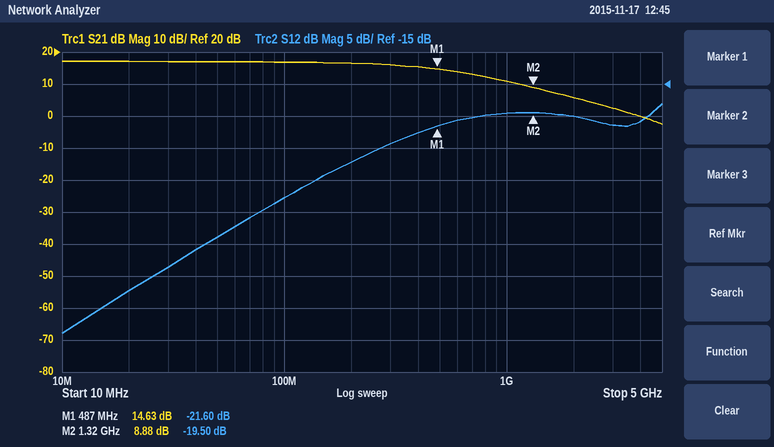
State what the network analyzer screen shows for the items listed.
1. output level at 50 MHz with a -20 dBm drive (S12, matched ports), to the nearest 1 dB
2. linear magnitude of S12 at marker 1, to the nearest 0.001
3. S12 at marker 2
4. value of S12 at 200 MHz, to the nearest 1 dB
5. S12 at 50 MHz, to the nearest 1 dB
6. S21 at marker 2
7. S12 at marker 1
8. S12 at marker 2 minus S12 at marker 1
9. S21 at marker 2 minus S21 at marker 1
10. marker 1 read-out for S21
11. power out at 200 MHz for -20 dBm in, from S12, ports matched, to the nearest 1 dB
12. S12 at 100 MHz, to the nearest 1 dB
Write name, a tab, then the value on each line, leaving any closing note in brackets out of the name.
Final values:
output level at 50 MHz with a -20 dBm drive (S12, matched ports), to the nearest 1 dB	-59 dBm
linear magnitude of S12 at marker 1, to the nearest 0.001	0.083
S12 at marker 2	-19.50 dB
value of S12 at 200 MHz, to the nearest 1 dB	-27 dB
S12 at 50 MHz, to the nearest 1 dB	-39 dB
S21 at marker 2	8.88 dB
S12 at marker 1	-21.60 dB
S12 at marker 2 minus S12 at marker 1	2.10 dB
S21 at marker 2 minus S21 at marker 1	-5.75 dB
marker 1 read-out for S21	14.63 dB
power out at 200 MHz for -20 dBm in, from S12, ports matched, to the nearest 1 dB	-47 dBm
S12 at 100 MHz, to the nearest 1 dB	-33 dB
